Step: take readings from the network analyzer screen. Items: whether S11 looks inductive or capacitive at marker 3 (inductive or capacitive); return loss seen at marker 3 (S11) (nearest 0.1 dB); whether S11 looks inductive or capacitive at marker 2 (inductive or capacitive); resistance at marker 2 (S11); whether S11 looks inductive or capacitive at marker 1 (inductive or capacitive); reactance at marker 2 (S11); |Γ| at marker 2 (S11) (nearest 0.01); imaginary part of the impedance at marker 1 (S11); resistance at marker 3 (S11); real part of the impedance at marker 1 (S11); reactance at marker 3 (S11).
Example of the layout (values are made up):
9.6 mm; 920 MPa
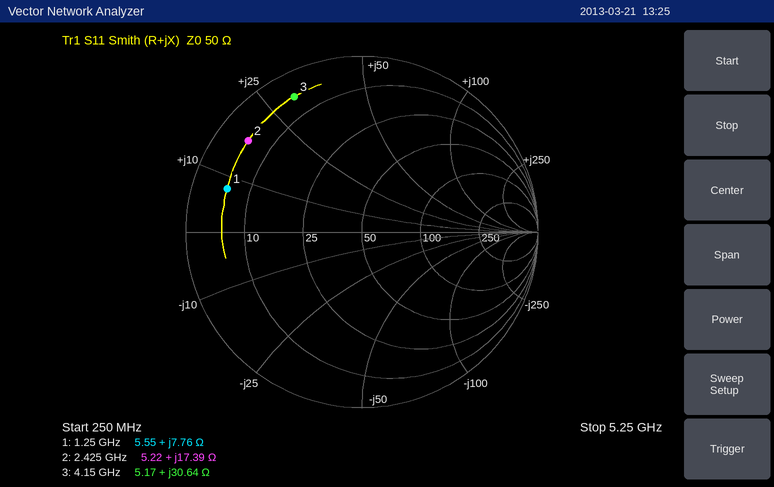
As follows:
inductive; 1.3 dB; inductive; 5.22 Ω; inductive; +17.39 Ω; 0.83; +7.76 Ω; 5.17 Ω; 5.55 Ω; +30.64 Ω
